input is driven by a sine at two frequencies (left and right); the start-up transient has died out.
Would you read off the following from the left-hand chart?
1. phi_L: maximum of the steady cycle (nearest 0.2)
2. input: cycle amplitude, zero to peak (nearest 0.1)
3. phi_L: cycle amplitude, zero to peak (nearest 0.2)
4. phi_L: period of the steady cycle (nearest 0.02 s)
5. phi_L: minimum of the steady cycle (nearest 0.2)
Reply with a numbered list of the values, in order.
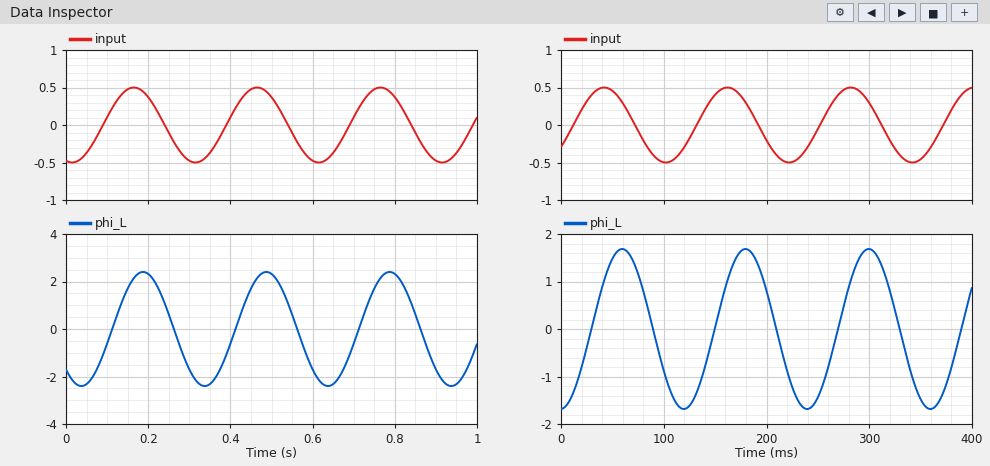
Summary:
1. 2.4
2. 0.5
3. 2.4
4. 0.30 s
5. -2.4
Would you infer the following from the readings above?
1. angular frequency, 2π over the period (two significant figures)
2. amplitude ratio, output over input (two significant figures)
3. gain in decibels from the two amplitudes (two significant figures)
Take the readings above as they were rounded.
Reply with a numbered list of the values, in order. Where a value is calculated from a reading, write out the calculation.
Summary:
1. 2π / 0.3 = 21 rad/s
2. 2.4 / 0.5 = 4.8
3. 20 log10(2.4 / 0.5) = 14 dB
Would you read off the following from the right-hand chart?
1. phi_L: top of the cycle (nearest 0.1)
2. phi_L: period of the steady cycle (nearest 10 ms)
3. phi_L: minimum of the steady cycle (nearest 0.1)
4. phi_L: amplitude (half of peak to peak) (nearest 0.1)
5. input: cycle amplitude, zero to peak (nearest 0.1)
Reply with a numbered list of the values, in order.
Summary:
1. 1.7
2. 120 ms
3. -1.7
4. 1.7
5. 0.5
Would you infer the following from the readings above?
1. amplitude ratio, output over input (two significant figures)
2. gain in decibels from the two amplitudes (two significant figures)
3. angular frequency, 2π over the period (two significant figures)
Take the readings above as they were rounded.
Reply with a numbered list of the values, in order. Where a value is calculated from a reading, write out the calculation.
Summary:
1. 1.7 / 0.5 = 3.4
2. 20 log10(1.7 / 0.5) = 11 dB
3. 2π / 120 = 0.052 rad/ms
